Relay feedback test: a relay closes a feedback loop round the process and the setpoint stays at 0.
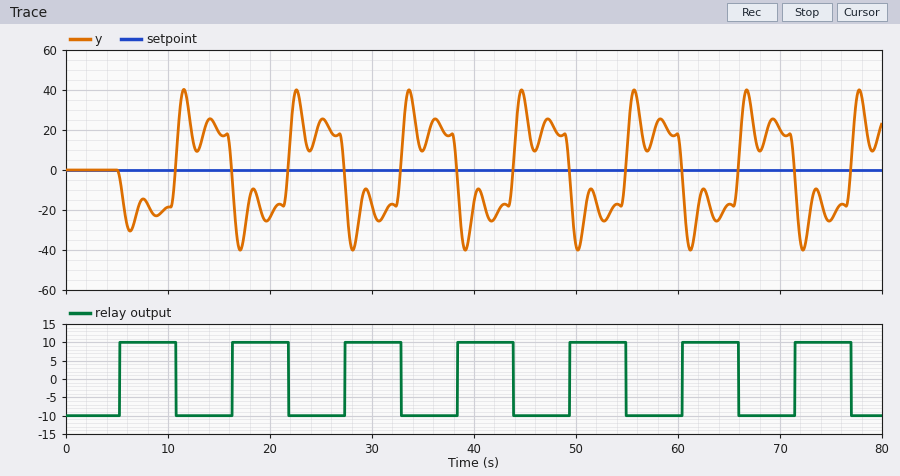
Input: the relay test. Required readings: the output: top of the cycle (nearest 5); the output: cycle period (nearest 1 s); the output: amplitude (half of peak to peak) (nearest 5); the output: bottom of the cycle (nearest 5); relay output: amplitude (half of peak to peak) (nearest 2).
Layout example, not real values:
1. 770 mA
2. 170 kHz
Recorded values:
1. 40
2. 11 s
3. 40
4. -40
5. 10
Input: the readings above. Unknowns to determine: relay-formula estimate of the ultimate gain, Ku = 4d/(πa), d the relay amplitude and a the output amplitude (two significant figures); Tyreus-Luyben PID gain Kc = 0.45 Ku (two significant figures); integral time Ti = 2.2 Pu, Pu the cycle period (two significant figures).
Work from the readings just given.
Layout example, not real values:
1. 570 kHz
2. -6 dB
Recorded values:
1. 0.32
2. 0.14
3. 24 s
